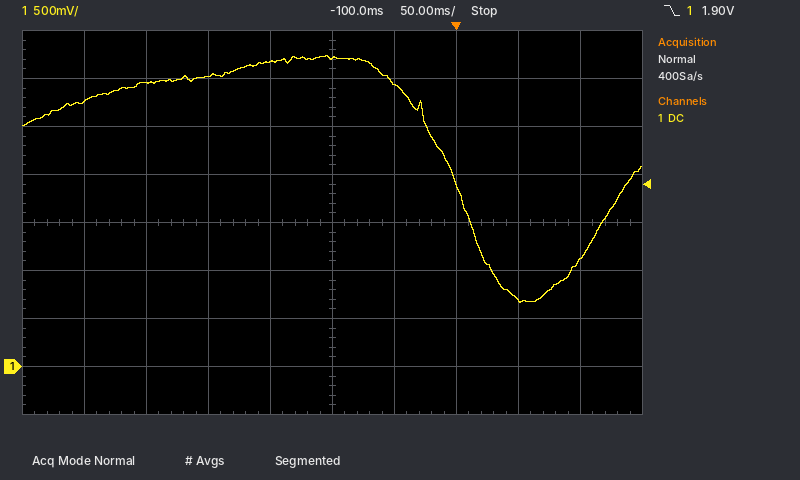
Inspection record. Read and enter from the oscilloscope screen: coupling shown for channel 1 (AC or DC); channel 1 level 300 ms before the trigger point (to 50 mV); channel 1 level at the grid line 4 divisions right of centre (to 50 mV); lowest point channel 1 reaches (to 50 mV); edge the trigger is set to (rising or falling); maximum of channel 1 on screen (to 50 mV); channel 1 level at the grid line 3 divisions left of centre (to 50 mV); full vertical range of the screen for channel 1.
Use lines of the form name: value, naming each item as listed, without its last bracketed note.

coupling shown for channel 1: DC
channel 1 level 300 ms before the trigger point: 2.75 V
channel 1 level at the grid line 4 divisions right of centre: 1.10 V
lowest point channel 1 reaches: 650 mV
edge the trigger is set to: falling
maximum of channel 1 on screen: 3.25 V
channel 1 level at the grid line 3 divisions left of centre: 2.95 V
full vertical range of the screen for channel 1: 4 V
